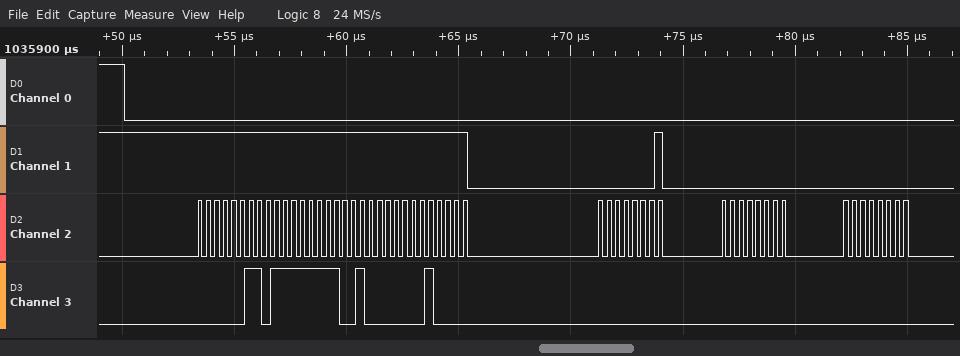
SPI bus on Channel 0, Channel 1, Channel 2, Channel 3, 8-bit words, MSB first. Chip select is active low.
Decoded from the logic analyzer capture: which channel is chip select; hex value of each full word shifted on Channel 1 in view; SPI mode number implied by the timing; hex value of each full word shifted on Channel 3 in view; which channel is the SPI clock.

Channel 0
FF, FF, FF, FF, 01, 00, 00
0
03, 7F, 90, 10, 00, 00, 00
Channel 2
